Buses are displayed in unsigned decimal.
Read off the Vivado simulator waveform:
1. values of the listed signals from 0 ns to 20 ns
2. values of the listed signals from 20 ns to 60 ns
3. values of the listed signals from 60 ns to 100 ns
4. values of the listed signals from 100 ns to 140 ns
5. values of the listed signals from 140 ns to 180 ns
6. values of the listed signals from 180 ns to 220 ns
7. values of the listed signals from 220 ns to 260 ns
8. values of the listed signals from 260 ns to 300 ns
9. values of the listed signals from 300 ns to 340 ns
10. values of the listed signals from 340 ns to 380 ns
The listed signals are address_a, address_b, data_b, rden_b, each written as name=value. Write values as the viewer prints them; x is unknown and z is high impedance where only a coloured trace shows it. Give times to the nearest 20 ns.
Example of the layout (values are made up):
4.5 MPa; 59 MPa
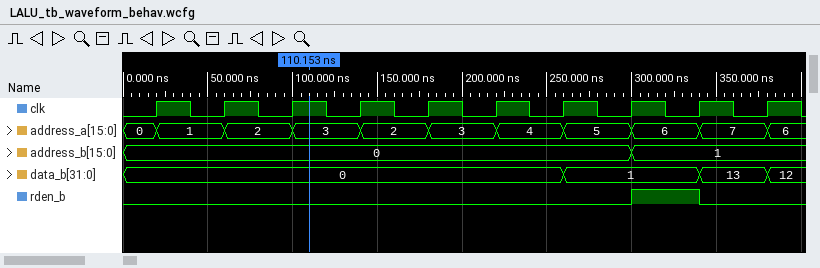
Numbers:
address_a=0, address_b=0, data_b=0, rden_b=0; address_a=1, address_b=0, data_b=0, rden_b=0; address_a=2, address_b=0, data_b=0, rden_b=0; address_a=3, address_b=0, data_b=0, rden_b=0; address_a=2, address_b=0, data_b=0, rden_b=0; address_a=3, address_b=0, data_b=0, rden_b=0; address_a=4, address_b=0, data_b=0, rden_b=0; address_a=5, address_b=0, data_b=1, rden_b=0; address_a=6, address_b=1, data_b=1, rden_b=1; address_a=7, address_b=1, data_b=13, rden_b=0
